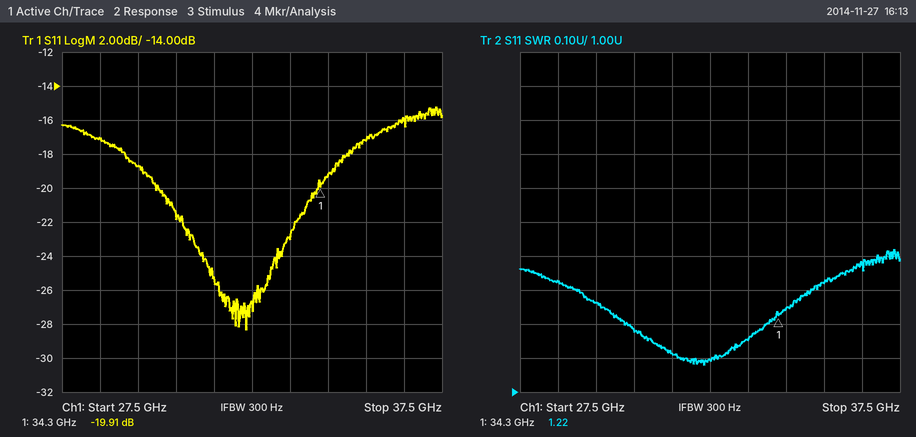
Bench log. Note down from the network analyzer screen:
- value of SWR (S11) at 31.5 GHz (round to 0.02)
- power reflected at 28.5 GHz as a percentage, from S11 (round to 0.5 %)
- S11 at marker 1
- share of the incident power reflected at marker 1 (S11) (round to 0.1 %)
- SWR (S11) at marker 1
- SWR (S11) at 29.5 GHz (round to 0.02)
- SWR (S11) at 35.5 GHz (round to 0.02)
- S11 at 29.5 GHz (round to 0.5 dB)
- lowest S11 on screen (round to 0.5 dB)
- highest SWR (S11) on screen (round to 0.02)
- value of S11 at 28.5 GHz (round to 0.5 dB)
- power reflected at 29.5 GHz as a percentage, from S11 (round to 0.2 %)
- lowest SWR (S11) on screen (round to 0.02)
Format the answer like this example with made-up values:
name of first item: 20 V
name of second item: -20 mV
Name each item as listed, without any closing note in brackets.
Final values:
value of SWR (S11) at 31.5 GHz: 1.12
power reflected at 28.5 GHz as a percentage, from S11: 2.0 %
S11 at marker 1: -19.91 dB
share of the incident power reflected at marker 1 (S11): 1.0 %
SWR (S11) at marker 1: 1.22
SWR (S11) at 29.5 GHz: 1.26
SWR (S11) at 35.5 GHz: 1.32
S11 at 29.5 GHz: -18.5 dB
lowest S11 on screen: -28.5 dB
highest SWR (S11) on screen: 1.42
value of S11 at 28.5 GHz: -17.0 dB
power reflected at 29.5 GHz as a percentage, from S11: 1.4 %
lowest SWR (S11) on screen: 1.08
